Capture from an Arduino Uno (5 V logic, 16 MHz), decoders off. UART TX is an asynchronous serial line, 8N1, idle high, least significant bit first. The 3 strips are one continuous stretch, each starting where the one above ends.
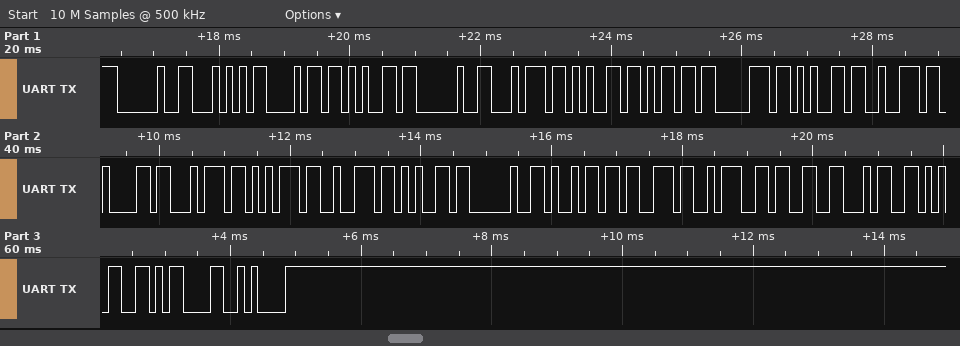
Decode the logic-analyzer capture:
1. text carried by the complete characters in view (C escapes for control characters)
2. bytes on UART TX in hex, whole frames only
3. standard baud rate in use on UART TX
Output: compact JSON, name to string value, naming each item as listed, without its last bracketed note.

{"text carried by the complete characters in view": "\" The temperature is:345\\r\\n\"", "bytes on UART TX in hex, whole frames only": "20 54 68 65 20 74 65 6D 70 65 72 61 74 75 72 65 20 69 73 3A 33 34 35 0D 0A", "standard baud rate in use on UART TX": "9600 baud"}
